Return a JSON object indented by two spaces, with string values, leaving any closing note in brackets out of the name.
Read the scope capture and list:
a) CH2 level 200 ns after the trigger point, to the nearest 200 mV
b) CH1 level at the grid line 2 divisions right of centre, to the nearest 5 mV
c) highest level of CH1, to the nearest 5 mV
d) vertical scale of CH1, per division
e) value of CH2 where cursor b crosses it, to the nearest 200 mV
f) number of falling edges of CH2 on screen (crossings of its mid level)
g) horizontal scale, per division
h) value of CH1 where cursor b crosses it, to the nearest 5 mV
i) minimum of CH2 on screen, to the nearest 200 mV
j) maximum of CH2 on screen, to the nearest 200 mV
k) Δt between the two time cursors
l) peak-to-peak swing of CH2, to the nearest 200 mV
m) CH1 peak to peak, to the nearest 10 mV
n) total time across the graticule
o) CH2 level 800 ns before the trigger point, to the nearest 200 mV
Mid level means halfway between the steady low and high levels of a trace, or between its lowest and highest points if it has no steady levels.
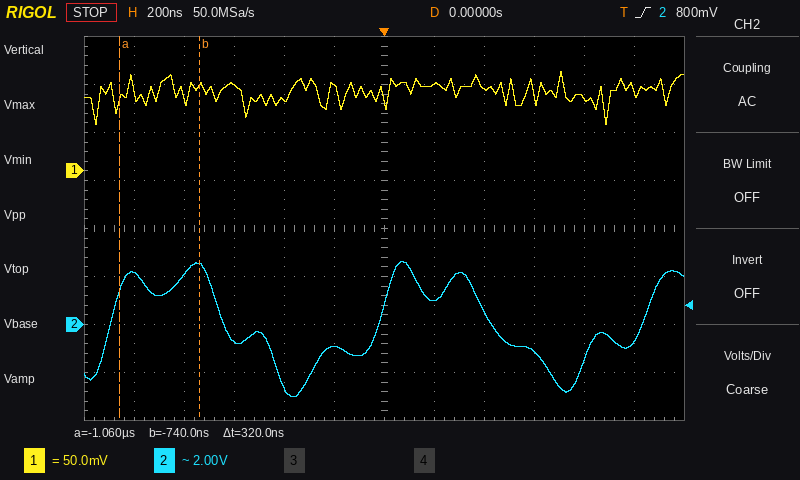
{
  "CH2 level 200 ns after the trigger point, to the nearest 200 mV": "1.0 V",
  "CH1 level at the grid line 2 divisions right of centre, to the nearest 5 mV": "85 mV",
  "highest level of CH1, to the nearest 5 mV": "105 mV",
  "vertical scale of CH1, per division": "50 mV",
  "value of CH2 where cursor b crosses it, to the nearest 200 mV": "2.4 V",
  "number of falling edges of CH2 on screen": "2",
  "horizontal scale, per division": "200 ns",
  "value of CH1 where cursor b crosses it, to the nearest 5 mV": "90 mV",
  "minimum of CH2 on screen, to the nearest 200 mV": "-3.0 V",
  "maximum of CH2 on screen, to the nearest 200 mV": "2.6 V",
  "Δt between the two time cursors": "320 ns",
  "peak-to-peak swing of CH2, to the nearest 200 mV": "5.6 V",
  "CH1 peak to peak, to the nearest 10 mV": "60 mV",
  "total time across the graticule": "2.4 µs",
  "CH2 level 800 ns before the trigger point, to the nearest 200 mV": "2.0 V"
}
